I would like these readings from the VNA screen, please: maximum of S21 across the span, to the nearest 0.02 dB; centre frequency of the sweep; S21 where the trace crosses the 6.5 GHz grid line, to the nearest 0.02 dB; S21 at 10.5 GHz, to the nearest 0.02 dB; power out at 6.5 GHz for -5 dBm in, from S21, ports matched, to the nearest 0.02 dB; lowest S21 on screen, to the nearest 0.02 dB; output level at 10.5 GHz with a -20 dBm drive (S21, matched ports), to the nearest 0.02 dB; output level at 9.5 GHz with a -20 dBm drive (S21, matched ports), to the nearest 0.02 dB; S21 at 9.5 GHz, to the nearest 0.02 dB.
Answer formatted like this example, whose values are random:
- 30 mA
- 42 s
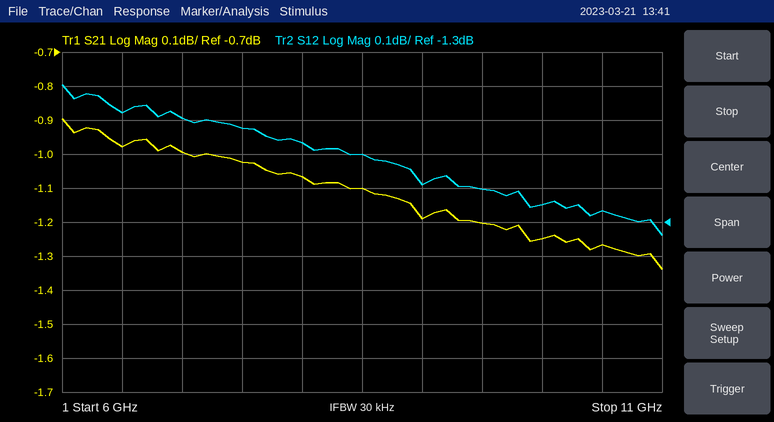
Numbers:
- -0.90 dB
- 8.5 GHz
- -0.98 dB
- -1.26 dB
- -5.98 dBm
- -1.34 dB
- -21.26 dBm
- -21.20 dBm
- -1.20 dB
